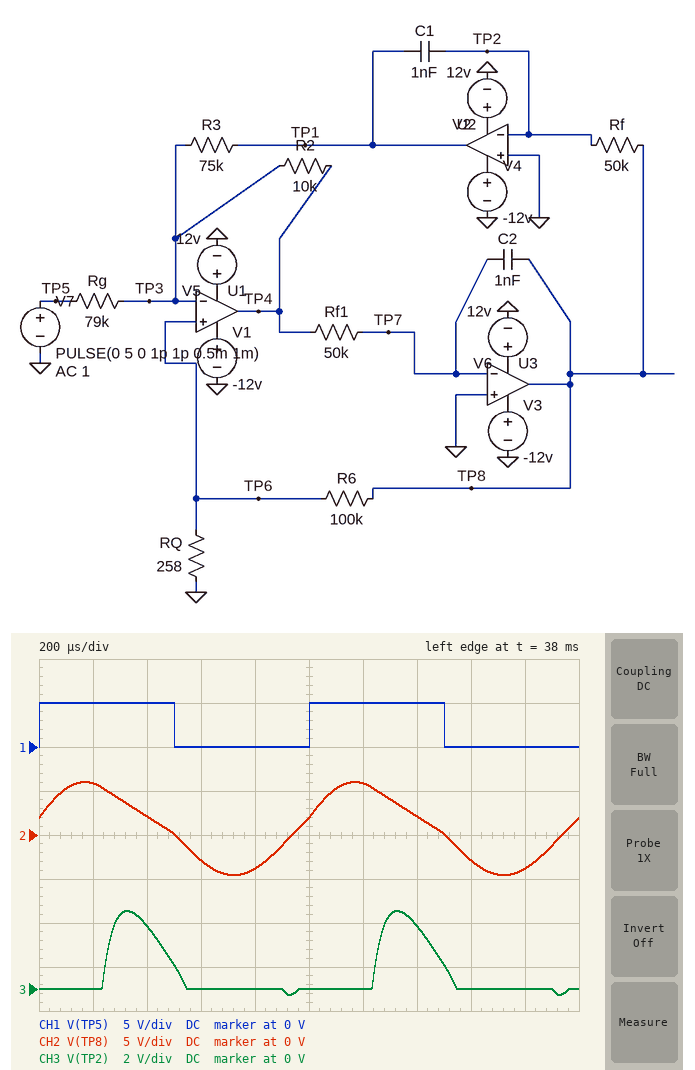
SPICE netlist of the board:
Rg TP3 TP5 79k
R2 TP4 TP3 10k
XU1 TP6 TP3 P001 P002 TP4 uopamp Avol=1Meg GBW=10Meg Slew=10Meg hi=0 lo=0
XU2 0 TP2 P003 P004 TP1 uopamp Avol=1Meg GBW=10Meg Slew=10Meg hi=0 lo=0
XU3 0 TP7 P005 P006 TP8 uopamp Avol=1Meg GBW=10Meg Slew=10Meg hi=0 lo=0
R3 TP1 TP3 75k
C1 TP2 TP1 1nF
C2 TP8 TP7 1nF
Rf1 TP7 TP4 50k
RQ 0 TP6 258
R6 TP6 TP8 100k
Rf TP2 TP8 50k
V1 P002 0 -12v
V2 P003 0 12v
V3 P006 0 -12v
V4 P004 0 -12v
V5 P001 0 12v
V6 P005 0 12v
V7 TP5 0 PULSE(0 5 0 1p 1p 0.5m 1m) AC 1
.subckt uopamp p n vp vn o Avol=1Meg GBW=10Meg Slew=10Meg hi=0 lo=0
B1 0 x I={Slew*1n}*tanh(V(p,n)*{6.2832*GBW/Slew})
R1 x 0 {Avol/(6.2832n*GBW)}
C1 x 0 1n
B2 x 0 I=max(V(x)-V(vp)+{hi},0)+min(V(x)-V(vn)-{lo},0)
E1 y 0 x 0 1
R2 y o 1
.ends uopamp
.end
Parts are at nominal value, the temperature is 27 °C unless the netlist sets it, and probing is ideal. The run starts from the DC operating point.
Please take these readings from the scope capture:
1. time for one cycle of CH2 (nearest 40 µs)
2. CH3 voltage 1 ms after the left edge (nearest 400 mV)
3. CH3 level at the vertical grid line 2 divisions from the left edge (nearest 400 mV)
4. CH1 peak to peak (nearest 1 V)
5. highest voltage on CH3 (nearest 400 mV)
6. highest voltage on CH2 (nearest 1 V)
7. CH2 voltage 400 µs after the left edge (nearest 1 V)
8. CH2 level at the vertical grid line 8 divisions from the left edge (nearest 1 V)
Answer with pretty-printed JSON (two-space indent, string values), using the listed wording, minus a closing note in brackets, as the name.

{
  "time for one cycle of CH2": "1.00 ms",
  "CH3 voltage 1 ms after the left edge": "0 V",
  "CH3 level at the vertical grid line 2 divisions from the left edge": "2.8 V",
  "CH1 peak to peak": "5 V",
  "highest voltage on CH3": "3.6 V",
  "highest voltage on CH2": "6 V",
  "CH2 voltage 400 µs after the left edge": "2 V",
  "CH2 level at the vertical grid line 8 divisions from the left edge": "-3 V"
}
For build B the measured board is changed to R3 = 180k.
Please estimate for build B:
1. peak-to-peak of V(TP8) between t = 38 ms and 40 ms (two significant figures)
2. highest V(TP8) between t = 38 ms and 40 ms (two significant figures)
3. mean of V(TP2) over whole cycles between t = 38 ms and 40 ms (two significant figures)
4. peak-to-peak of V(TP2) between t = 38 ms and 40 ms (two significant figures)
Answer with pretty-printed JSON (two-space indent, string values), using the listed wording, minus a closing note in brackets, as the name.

{
  "peak-to-peak of V(TP8) between t = 38 ms and 40 ms": "5.8 V",
  "highest V(TP8) between t = 38 ms and 40 ms": "3.1 V",
  "mean of V(TP2) over whole cycles between t = 38 ms and 40 ms": "180 mV",
  "peak-to-peak of V(TP2) between t = 38 ms and 40 ms": "1.3 V"
}
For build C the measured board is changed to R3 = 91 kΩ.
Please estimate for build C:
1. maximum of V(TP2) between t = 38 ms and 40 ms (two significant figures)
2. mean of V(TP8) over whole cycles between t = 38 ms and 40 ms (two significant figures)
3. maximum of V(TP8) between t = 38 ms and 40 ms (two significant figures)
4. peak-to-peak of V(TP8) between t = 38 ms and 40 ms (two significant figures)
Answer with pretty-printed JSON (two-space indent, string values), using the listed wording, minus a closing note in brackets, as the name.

{
  "maximum of V(TP2) between t = 38 ms and 40 ms": "3.8 V",
  "mean of V(TP8) over whole cycles between t = 38 ms and 40 ms": "770 mV",
  "maximum of V(TP8) between t = 38 ms and 40 ms": "5.7 V",
  "peak-to-peak of V(TP8) between t = 38 ms and 40 ms": "9.8 V"
}
